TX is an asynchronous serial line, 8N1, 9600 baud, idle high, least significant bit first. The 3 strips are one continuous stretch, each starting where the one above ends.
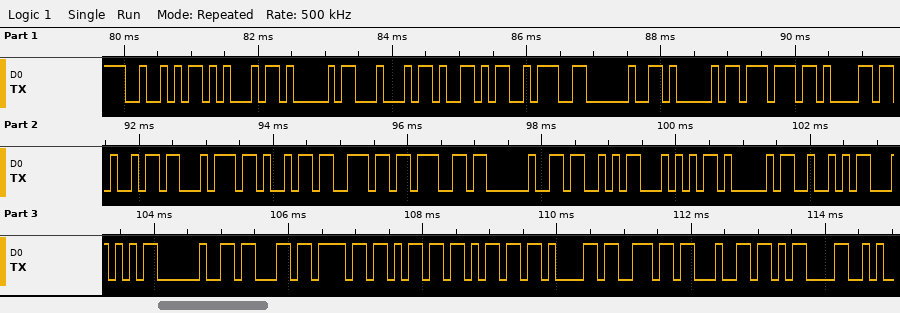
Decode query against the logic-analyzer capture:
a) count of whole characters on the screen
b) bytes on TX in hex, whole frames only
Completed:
30
52 45 41 44 59 3A 20 41 77 61 69 74 69 6E 67 20 53 54 41 52 54 20 63 6F 6D 6D 61 6E 64 0D
